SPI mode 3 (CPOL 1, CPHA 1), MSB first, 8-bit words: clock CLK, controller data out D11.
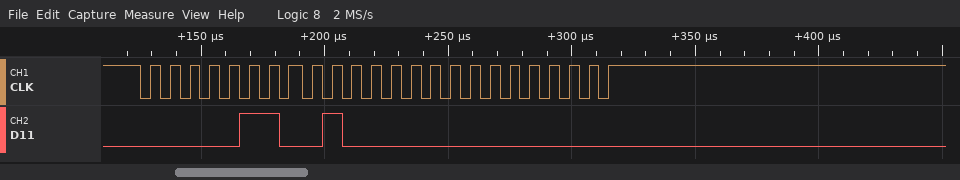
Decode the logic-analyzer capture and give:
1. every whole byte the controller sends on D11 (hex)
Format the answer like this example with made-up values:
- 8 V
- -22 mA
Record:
- 06 40 00
